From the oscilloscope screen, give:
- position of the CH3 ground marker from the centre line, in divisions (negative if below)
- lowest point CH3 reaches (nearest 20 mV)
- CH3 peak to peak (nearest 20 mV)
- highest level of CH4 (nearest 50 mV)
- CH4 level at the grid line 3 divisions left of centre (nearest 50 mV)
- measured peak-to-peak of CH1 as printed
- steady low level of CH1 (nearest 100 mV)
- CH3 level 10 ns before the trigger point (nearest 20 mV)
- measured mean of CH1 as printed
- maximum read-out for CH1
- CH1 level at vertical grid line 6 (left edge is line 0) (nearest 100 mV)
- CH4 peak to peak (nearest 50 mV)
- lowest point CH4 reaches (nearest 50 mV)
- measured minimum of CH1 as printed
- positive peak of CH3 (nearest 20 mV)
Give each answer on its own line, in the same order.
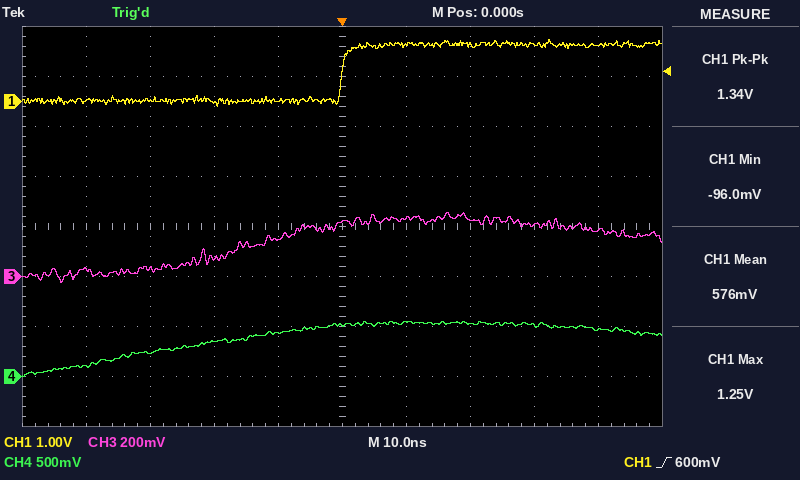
-1.0 div
-20 mV
280 mV
550 mV
250 mV
1.34 V
0.0 V
140 mV
576 mV
1.25 V
1.1 V
550 mV
0 mV
-96.0 mV
260 mV
